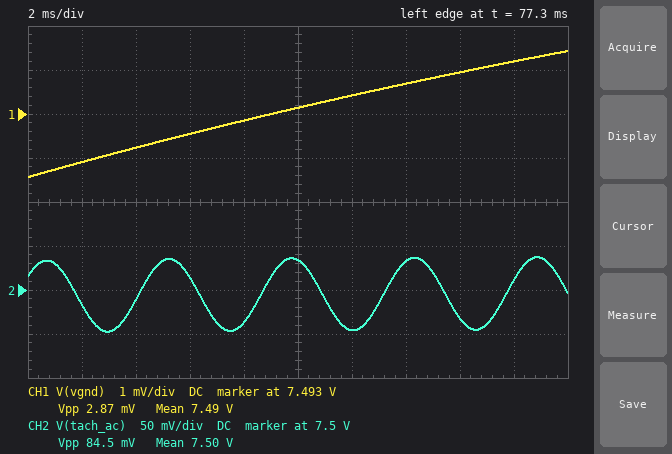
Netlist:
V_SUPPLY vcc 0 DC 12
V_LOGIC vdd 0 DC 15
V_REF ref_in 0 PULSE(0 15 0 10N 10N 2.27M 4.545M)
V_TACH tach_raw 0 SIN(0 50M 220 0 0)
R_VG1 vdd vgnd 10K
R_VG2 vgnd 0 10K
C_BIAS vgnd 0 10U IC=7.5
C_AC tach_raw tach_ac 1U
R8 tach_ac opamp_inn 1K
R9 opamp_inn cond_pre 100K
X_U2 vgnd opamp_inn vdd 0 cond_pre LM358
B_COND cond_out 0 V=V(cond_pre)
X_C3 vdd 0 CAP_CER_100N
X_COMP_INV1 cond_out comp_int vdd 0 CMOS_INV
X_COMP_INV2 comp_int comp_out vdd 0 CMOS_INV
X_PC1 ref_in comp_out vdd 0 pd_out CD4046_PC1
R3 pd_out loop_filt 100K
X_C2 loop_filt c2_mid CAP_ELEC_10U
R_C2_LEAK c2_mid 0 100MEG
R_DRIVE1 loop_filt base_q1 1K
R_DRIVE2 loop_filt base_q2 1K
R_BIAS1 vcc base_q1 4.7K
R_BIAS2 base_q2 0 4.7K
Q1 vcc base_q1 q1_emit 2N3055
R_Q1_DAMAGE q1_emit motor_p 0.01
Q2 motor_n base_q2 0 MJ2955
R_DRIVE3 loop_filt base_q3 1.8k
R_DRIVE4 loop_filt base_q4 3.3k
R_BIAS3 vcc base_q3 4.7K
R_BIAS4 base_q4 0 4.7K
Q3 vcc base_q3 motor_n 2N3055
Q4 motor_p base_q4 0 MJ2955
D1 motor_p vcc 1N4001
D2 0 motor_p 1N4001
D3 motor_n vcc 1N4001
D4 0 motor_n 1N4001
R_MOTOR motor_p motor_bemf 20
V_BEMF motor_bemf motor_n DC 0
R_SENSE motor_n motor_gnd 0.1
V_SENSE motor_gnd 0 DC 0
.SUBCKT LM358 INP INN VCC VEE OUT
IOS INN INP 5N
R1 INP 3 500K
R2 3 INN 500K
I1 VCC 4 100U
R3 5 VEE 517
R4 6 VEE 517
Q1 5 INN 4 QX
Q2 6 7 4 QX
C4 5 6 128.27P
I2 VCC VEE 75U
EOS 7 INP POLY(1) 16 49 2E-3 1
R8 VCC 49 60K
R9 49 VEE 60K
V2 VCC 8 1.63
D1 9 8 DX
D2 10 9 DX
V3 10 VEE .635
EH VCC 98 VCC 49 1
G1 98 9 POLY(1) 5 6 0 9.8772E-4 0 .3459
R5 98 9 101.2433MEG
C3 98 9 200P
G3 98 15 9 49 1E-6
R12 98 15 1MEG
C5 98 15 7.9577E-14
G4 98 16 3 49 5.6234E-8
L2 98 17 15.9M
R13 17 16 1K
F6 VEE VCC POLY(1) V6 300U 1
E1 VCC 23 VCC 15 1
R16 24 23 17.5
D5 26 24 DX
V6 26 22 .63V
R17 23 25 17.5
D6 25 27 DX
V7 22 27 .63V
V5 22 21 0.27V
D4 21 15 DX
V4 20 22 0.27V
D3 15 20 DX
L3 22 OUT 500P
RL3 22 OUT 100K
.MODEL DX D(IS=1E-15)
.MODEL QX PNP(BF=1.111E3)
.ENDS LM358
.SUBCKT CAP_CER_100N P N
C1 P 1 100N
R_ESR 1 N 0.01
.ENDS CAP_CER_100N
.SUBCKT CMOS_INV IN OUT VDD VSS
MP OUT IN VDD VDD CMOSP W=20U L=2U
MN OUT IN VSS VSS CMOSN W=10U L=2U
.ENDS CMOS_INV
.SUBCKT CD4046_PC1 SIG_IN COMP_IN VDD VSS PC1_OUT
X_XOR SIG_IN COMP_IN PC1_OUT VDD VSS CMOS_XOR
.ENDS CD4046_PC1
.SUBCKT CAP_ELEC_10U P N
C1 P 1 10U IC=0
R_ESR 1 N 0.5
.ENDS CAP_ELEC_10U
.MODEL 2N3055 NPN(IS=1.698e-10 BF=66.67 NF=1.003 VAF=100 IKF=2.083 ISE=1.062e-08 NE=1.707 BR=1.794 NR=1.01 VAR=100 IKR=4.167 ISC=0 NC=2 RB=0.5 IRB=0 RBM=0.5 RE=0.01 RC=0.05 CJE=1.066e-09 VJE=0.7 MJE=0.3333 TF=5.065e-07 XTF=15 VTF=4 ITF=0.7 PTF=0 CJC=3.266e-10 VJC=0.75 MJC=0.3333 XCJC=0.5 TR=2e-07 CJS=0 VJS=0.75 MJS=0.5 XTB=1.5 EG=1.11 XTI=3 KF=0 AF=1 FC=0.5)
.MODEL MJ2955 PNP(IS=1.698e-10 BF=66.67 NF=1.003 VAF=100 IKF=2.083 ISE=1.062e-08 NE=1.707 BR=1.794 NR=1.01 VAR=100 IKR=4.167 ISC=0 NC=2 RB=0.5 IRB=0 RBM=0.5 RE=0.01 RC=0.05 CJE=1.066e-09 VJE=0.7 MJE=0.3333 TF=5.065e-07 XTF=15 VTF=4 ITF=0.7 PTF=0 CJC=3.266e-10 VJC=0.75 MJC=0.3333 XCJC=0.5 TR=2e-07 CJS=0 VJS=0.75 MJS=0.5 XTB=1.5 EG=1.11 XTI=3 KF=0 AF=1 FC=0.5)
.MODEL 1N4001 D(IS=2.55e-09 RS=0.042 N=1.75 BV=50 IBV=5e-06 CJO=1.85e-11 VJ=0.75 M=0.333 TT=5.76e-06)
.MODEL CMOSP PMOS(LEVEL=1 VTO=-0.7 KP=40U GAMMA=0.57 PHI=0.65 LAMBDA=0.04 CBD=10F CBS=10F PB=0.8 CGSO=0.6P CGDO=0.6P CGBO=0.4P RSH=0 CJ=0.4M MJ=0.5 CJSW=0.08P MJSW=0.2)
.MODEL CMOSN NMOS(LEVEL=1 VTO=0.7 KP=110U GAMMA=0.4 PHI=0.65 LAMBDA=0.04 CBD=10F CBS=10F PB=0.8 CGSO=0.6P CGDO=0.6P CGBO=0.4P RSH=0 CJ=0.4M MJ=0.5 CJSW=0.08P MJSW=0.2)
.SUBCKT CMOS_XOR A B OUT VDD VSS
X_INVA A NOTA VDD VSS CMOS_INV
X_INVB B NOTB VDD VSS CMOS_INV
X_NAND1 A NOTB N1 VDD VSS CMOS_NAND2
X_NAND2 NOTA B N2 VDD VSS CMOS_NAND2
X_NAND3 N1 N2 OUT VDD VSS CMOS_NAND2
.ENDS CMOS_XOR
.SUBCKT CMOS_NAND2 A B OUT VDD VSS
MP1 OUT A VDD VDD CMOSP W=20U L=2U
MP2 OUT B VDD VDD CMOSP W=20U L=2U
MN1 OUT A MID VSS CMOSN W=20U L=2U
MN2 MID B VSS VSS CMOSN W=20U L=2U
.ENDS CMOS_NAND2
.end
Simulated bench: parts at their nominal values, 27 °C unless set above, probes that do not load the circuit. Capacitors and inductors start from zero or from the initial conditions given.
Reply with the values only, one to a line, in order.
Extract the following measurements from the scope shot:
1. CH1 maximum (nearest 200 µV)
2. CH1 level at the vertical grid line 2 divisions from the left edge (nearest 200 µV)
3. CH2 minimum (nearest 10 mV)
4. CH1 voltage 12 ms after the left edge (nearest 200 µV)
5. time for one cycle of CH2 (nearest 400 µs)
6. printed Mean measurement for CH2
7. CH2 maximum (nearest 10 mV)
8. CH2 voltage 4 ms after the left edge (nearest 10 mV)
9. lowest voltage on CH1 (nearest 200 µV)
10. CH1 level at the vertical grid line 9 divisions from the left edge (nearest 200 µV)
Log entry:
7.4944 V
7.4922 V
7.45 V
7.4934 V
4.4 ms
7.50 V
7.54 V
7.49 V
7.4916 V
7.4942 V
